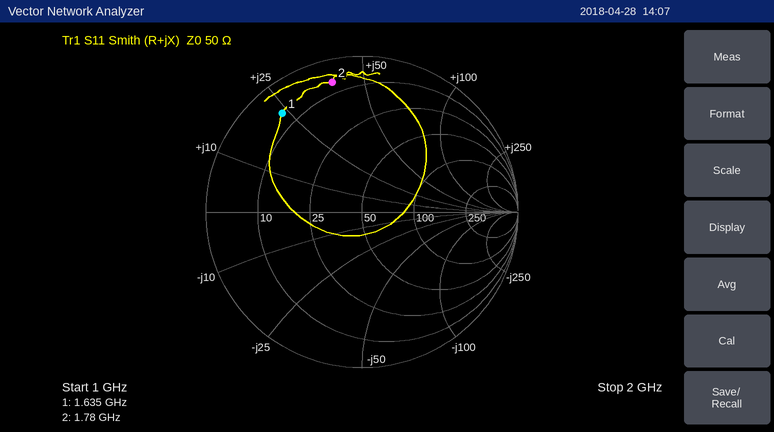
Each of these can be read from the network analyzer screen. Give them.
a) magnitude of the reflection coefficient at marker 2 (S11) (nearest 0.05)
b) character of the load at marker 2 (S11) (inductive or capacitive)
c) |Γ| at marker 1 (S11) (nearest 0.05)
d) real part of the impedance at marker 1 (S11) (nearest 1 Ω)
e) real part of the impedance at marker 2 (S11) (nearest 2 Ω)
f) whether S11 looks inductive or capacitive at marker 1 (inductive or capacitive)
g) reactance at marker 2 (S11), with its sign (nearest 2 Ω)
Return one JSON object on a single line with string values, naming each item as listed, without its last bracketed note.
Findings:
{"magnitude of the reflection coefficient at marker 2 (S11)": "0.85", "character of the load at marker 2 (S11)": "inductive", "|Γ| at marker 1 (S11)": "0.80", "real part of the impedance at marker 1 (S11)": "6 Ω", "real part of the impedance at marker 2 (S11)": "6 Ω", "whether S11 looks inductive or capacitive at marker 1": "inductive", "reactance at marker 2 (S11), with its sign": "+40 Ω"}
